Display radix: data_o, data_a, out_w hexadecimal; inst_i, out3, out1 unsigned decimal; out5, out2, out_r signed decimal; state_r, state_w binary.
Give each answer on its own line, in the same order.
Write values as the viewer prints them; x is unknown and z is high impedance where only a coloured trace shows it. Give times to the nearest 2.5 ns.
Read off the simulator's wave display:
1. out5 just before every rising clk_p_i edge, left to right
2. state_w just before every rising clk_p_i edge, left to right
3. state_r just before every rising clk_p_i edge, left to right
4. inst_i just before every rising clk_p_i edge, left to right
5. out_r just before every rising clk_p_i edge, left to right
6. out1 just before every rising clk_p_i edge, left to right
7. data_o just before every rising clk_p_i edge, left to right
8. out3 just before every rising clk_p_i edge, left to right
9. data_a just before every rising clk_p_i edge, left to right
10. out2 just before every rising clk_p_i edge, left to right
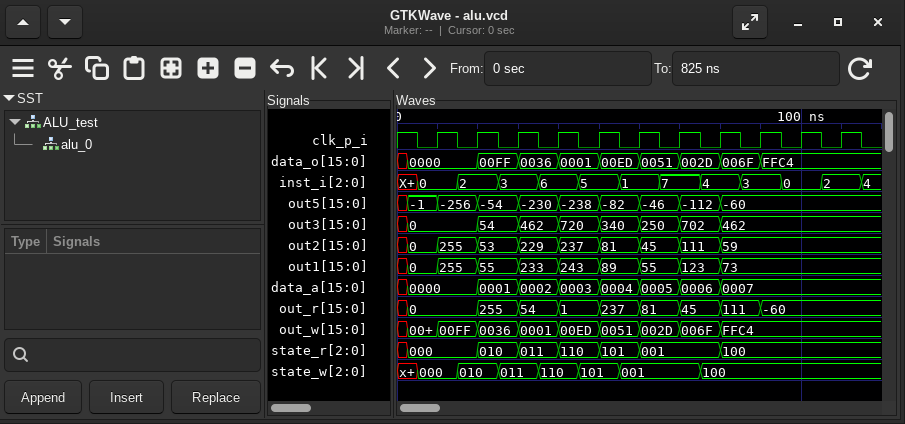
-1, -256, -54, -230, -238, -82, -46, -112, -60, -60, -60
000, 010, 011, 110, 101, 001, 001, 100, 100, 100, 100
000, 000, 010, 011, 110, 101, 001, 001, 100, 100, 100
0, 2, 3, 6, 5, 1, 7, 4, 3, 0, 2
0, 0, 255, 54, 1, 237, 81, 45, 111, -60, -60
0, 255, 55, 233, 243, 89, 55, 123, 73, 73, 73
0000, 0000, 00FF, 0036, 0001, 00ED, 0051, 002D, 006F, FFC4, FFC4
0, 0, 54, 462, 720, 340, 250, 702, 462, 462, 462
0000, 0000, 0001, 0002, 0003, 0004, 0005, 0006, 0007, 0007, 0007
0, 255, 53, 229, 237, 81, 45, 111, 59, 59, 59
